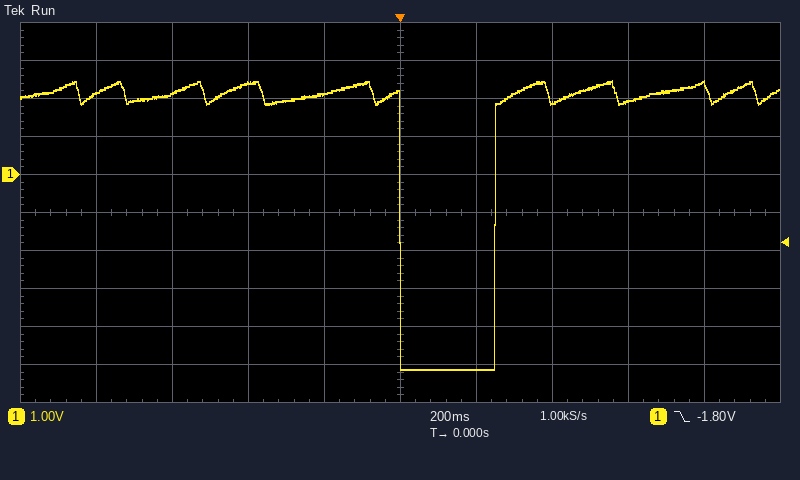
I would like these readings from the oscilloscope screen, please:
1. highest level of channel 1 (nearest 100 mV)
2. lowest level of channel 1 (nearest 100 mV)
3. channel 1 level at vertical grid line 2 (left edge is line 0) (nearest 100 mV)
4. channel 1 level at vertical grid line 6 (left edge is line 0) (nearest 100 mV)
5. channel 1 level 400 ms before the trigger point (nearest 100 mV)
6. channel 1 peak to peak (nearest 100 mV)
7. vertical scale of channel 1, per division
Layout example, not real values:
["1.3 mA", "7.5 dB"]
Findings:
["2.5 V", "-5.1 V", "2.1 V", "-5.1 V", "2.4 V", "7.6 V", "1 V"]
